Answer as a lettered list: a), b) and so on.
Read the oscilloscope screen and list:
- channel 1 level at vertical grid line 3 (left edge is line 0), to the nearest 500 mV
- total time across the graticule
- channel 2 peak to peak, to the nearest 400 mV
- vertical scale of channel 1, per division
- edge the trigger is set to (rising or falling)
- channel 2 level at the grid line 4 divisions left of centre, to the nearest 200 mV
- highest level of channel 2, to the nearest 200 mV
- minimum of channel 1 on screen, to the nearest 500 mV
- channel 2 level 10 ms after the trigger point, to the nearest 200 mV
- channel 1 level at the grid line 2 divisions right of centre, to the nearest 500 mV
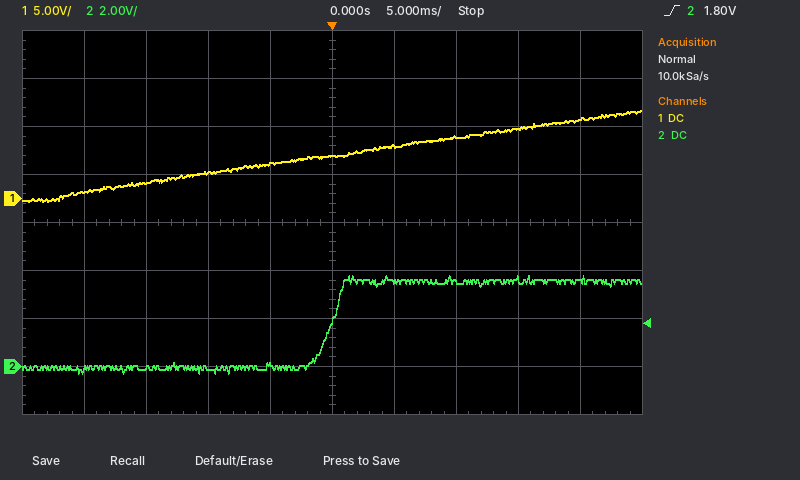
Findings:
a) 2.5 V
b) 50 ms
c) 4.0 V
d) 5 V
e) rising
f) -200 mV
g) 3.8 V
h) -500 mV
i) 3.6 V
j) 6.5 V
